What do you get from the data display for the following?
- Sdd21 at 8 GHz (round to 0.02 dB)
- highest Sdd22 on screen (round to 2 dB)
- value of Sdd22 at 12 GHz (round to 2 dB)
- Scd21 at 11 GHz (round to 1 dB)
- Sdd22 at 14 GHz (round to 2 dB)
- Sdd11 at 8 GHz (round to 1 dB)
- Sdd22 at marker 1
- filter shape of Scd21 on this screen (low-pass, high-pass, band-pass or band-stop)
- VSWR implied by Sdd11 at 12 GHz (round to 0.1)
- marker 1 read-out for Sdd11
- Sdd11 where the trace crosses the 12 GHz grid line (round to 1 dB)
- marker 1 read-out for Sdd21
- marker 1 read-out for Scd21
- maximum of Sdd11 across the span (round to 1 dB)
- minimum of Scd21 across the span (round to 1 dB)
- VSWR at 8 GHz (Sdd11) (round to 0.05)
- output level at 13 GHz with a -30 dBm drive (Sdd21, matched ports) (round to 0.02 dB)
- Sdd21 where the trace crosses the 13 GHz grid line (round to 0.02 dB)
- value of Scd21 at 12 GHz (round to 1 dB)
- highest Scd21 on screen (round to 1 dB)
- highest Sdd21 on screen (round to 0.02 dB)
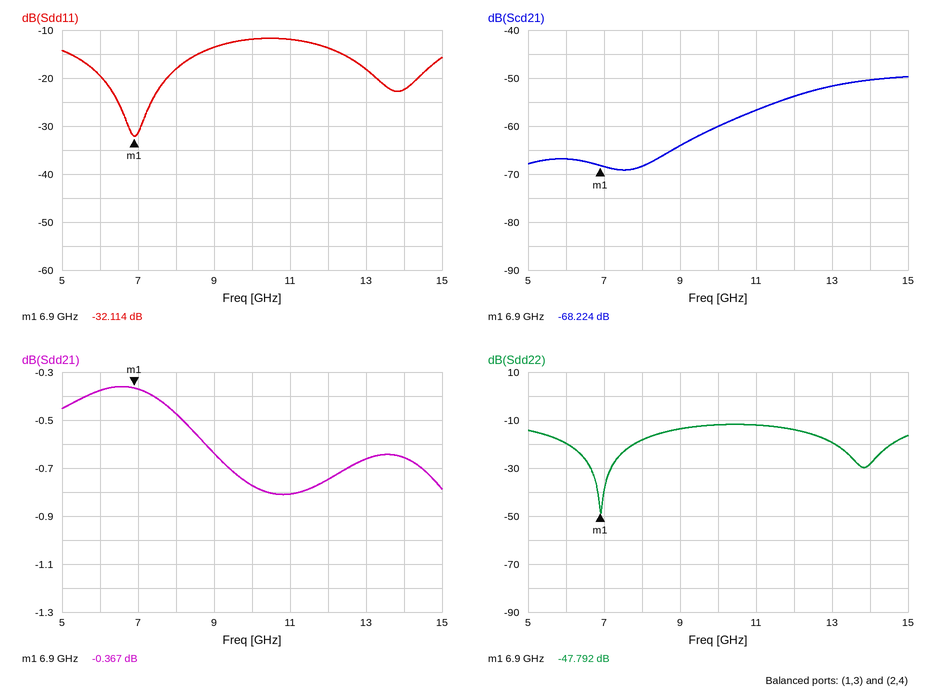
-0.48 dB
-12 dB
-14 dB
-57 dB
-28 dB
-18 dB
-47.792 dB
high-pass
1.5
-32.114 dB
-14 dB
-0.367 dB
-68.224 dB
-12 dB
-69 dB
1.30
-30.66 dBm
-0.66 dB
-54 dB
-50 dB
-0.36 dB
